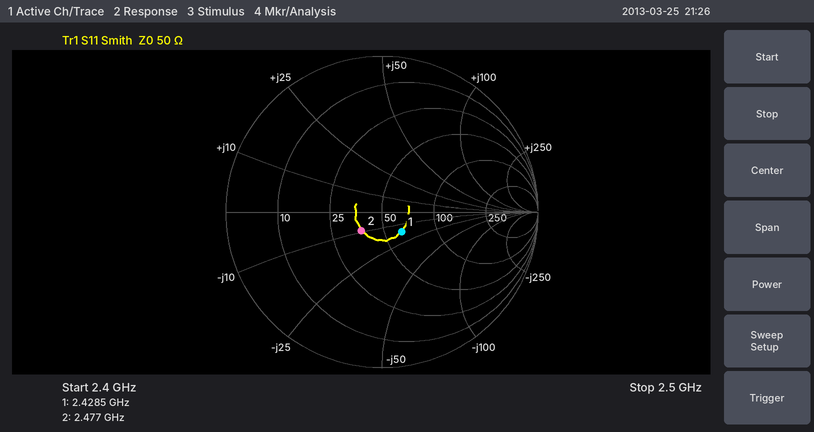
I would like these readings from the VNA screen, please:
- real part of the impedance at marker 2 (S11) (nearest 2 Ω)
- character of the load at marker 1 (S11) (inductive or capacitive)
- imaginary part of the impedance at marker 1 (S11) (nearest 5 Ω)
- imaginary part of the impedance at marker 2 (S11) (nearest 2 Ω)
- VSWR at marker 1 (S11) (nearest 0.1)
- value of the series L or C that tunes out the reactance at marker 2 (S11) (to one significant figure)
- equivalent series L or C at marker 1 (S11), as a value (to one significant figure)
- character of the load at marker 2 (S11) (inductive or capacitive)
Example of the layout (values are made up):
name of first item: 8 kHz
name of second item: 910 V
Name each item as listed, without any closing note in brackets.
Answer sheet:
real part of the impedance at marker 2 (S11): 38 Ω
character of the load at marker 1 (S11): capacitive
imaginary part of the impedance at marker 1 (S11): -15 Ω
imaginary part of the impedance at marker 2 (S11): -10 Ω
VSWR at marker 1 (S11): 1.4
value of the series L or C that tunes out the reactance at marker 2 (S11): 600 pH
equivalent series L or C at marker 1 (S11), as a value: 4 pF
character of the load at marker 2 (S11): capacitive
